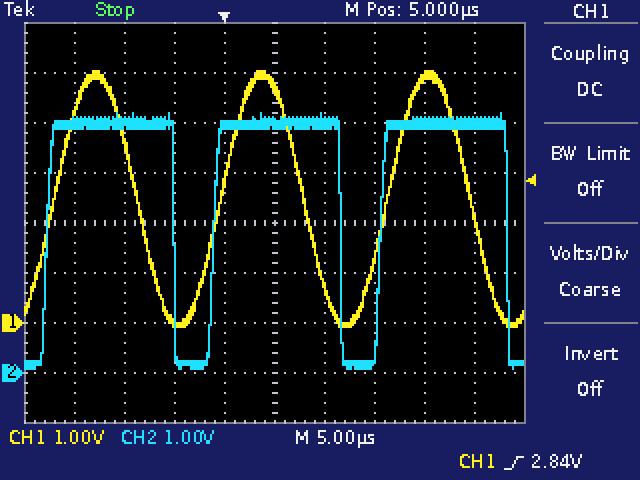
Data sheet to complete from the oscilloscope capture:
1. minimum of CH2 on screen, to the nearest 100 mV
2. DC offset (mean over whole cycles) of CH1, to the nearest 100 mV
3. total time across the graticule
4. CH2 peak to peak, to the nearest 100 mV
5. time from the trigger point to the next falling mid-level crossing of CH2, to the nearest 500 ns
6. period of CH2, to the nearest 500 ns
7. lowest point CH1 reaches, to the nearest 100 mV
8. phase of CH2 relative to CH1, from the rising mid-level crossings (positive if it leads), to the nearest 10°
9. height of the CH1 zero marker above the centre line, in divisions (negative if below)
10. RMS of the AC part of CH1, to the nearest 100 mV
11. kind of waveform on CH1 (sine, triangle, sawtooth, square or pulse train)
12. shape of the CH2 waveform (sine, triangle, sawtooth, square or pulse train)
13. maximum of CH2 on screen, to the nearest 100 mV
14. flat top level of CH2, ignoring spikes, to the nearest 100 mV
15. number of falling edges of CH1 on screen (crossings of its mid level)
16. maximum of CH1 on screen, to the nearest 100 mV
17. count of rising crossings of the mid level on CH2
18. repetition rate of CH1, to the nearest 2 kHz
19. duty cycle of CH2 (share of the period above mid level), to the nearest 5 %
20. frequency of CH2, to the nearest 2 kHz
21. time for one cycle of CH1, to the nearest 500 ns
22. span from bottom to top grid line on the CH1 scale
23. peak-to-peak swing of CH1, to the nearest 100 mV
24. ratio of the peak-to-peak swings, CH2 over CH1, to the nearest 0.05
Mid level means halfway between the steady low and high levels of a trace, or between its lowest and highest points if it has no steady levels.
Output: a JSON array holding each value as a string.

["100 mV", "2.5 V", "50 µs", "5.1 V", "11.5 µs", "16.5 µs", "-100 mV", "+20°", "-2.0 div", "1.8 V", "sine", "pulse train", "5.2 V", "5.0 V", "3", "5.0 V", "3", "60 kHz", "75 %", "60 kHz", "16.5 µs", "8 V", "5.1 V", "1.00"]
